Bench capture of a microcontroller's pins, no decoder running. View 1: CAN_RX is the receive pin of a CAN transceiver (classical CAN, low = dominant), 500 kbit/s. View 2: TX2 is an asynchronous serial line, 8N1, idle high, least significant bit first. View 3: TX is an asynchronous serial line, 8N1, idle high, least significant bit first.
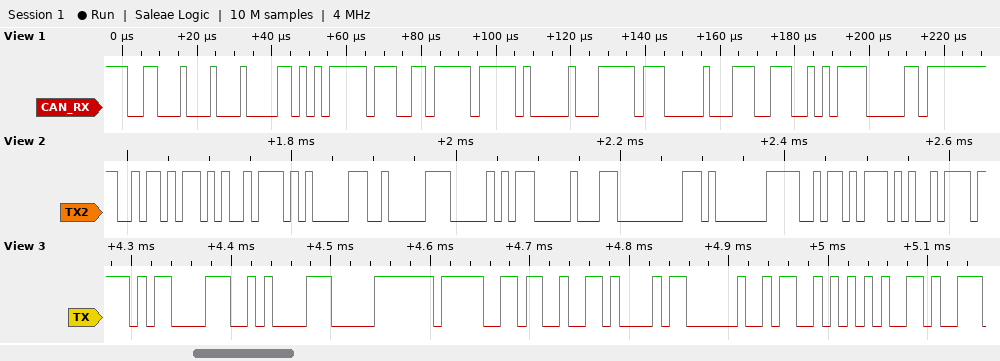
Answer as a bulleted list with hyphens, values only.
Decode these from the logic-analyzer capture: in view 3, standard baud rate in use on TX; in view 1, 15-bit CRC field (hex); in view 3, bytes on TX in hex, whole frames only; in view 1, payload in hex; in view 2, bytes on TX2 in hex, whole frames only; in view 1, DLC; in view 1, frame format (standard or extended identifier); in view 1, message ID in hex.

- 115200 baud
- 0x15E0
- 0D 0A F0 9F 93 A1 20 53 65
- 6A FF 37 FF 00 FF 00 E7
- 5A A5 05 82 50 10 00 01 5A A5
- 8
- standard
- 0x311
